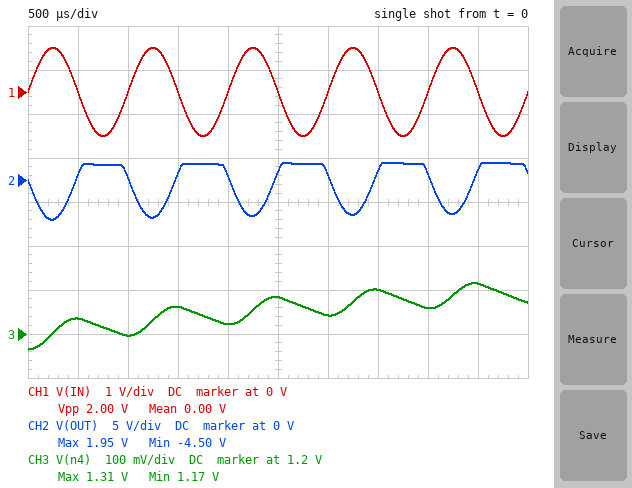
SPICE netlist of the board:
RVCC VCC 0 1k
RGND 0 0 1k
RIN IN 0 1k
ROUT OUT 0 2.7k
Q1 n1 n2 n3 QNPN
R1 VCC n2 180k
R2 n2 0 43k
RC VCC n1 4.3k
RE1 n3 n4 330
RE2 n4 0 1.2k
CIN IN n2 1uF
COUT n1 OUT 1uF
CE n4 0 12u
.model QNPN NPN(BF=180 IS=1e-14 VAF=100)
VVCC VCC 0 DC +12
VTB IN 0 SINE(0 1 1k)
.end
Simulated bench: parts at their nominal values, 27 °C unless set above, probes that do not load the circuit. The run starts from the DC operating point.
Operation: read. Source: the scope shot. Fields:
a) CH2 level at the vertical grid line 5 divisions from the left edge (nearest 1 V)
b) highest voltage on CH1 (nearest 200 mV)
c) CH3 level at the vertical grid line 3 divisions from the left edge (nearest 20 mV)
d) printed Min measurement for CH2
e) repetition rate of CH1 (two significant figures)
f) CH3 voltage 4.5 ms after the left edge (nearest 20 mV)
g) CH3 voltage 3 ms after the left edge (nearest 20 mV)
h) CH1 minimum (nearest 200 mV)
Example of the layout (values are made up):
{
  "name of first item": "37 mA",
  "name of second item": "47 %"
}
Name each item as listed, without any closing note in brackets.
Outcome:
{
  "CH2 level at the vertical grid line 5 divisions from the left edge": "1 V",
  "highest voltage on CH1": "1.0 V",
  "CH3 level at the vertical grid line 3 divisions from the left edge": "1.26 V",
  "printed Min measurement for CH2": "-4.50 V",
  "repetition rate of CH1": "1.0 kHz",
  "CH3 voltage 4.5 ms after the left edge": "1.32 V",
  "CH3 voltage 3 ms after the left edge": "1.24 V",
  "CH1 minimum": "-1.0 V"
}
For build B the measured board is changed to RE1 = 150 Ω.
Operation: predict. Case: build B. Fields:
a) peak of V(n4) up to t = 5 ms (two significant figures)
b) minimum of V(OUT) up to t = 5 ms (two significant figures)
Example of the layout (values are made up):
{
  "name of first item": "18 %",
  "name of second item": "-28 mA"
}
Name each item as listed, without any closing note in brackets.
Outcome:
{
  "peak of V(n4) up to t = 5 ms": "1.4 V",
  "minimum of V(OUT) up to t = 5 ms": "-5.2 V"
}
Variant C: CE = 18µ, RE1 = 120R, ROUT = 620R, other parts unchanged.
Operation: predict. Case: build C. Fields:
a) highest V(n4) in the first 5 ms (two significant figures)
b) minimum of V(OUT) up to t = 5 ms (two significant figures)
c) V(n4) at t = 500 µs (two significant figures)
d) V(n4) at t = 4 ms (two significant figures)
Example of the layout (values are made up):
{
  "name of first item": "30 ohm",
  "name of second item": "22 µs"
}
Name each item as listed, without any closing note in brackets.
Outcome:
{
  "highest V(n4) in the first 5 ms": "1.6 V",
  "minimum of V(OUT) up to t = 5 ms": "-3.8 V",
  "V(n4) at t = 500 µs": "1.4 V",
  "V(n4) at t = 4 ms": "1.5 V"
}
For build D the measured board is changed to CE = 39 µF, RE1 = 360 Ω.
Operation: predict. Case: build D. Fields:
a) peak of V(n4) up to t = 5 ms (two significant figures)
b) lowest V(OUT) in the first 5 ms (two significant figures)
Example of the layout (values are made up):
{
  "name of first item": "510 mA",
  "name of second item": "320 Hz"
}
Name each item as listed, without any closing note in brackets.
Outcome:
{
  "peak of V(n4) up to t = 5 ms": "1.2 V",
  "lowest V(OUT) in the first 5 ms": "-4.2 V"
}
